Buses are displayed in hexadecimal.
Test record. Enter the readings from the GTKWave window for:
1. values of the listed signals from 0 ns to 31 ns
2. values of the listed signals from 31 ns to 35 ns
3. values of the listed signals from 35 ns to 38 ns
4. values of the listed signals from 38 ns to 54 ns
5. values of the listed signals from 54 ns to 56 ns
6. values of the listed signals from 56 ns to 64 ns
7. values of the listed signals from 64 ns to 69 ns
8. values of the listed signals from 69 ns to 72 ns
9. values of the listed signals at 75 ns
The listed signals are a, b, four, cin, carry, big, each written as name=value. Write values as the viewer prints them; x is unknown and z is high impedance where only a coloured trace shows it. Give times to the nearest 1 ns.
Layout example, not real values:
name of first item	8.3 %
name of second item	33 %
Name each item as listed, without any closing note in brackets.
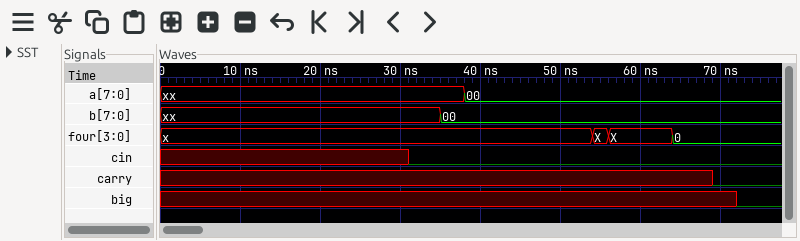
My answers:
values of the listed signals from 0 ns to 31 ns	a=xx, b=xx, four=x, cin=x, carry=x, big=x
values of the listed signals from 31 ns to 35 ns	a=xx, b=xx, four=x, cin=0, carry=x, big=x
values of the listed signals from 35 ns to 38 ns	a=xx, b=00, four=x, cin=0, carry=x, big=x
values of the listed signals from 38 ns to 54 ns	a=00, b=00, four=x, cin=0, carry=x, big=x
values of the listed signals from 54 ns to 56 ns	a=00, b=00, four=X, cin=0, carry=x, big=x
values of the listed signals from 56 ns to 64 ns	a=00, b=00, four=X, cin=0, carry=x, big=x
values of the listed signals from 64 ns to 69 ns	a=00, b=00, four=0, cin=0, carry=x, big=x
values of the listed signals from 69 ns to 72 ns	a=00, b=00, four=0, cin=0, carry=0, big=x
values of the listed signals at 75 ns	a=00, b=00, four=0, cin=0, carry=0, big=0
